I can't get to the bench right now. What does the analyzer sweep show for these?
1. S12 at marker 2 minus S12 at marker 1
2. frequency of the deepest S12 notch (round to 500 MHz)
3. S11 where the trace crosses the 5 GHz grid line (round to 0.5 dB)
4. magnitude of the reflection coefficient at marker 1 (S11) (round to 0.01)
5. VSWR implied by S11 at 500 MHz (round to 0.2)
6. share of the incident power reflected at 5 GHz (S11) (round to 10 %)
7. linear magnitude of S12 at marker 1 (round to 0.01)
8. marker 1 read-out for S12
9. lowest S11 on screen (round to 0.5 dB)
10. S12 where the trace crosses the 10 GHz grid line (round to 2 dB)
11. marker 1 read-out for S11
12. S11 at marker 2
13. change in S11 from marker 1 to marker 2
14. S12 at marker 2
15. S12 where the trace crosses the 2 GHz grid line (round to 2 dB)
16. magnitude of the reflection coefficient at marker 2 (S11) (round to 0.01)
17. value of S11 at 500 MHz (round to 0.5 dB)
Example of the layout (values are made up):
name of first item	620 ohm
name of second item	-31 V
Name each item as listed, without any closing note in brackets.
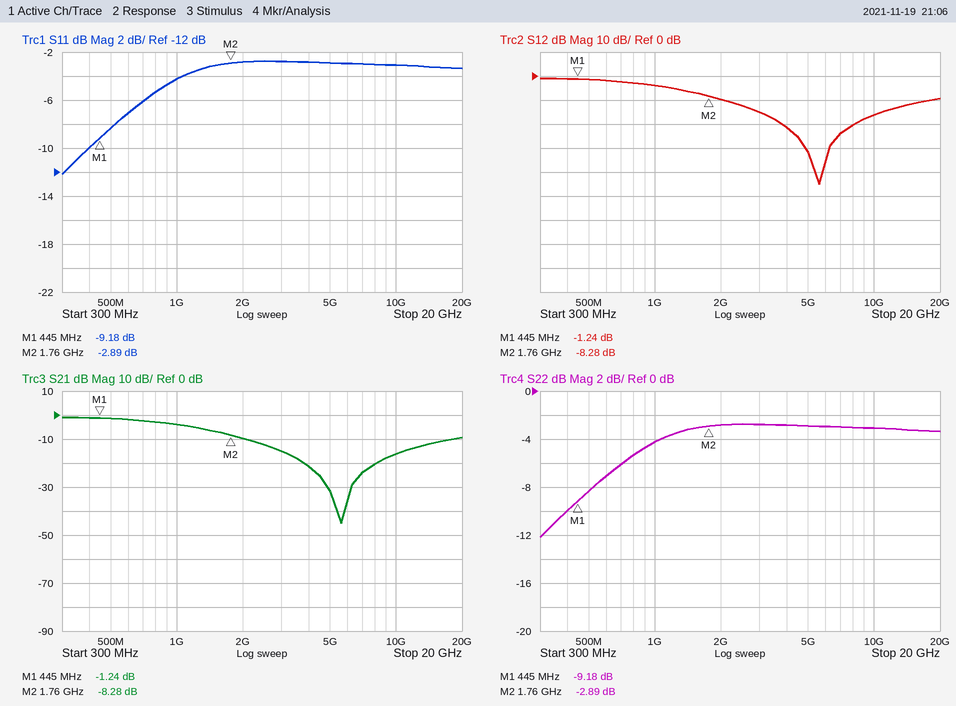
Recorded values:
S12 at marker 2 minus S12 at marker 1	-7.04 dB
frequency of the deepest S12 notch	5.5 GHz
S11 where the trace crosses the 5 GHz grid line	-3.0 dB
magnitude of the reflection coefficient at marker 1 (S11)	0.35
VSWR implied by S11 at 500 MHz	2.2
share of the incident power reflected at 5 GHz (S11)	50 %
linear magnitude of S12 at marker 1	0.87
marker 1 read-out for S12	-1.24 dB
lowest S11 on screen	-12.0 dB
S12 where the trace crosses the 10 GHz grid line	-16 dB
marker 1 read-out for S11	-9.18 dB
S11 at marker 2	-2.89 dB
change in S11 from marker 1 to marker 2	6.29 dB
S12 at marker 2	-8.28 dB
S12 where the trace crosses the 2 GHz grid line	-10 dB
magnitude of the reflection coefficient at marker 2 (S11)	0.72
value of S11 at 500 MHz	-8.5 dB
